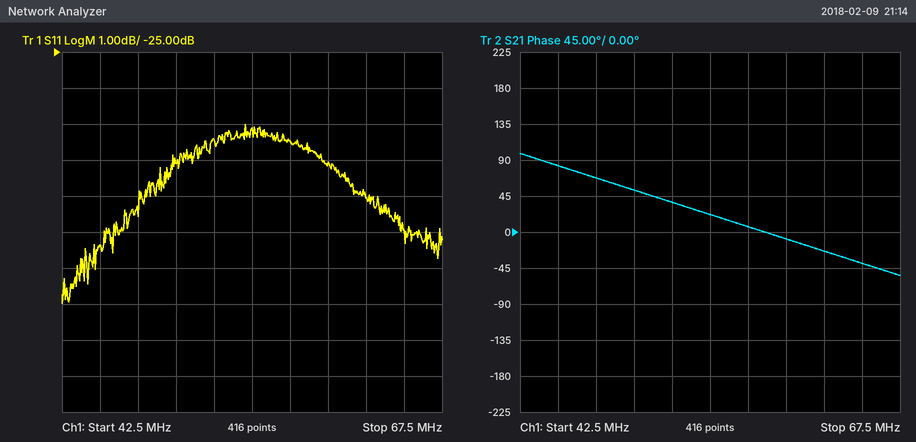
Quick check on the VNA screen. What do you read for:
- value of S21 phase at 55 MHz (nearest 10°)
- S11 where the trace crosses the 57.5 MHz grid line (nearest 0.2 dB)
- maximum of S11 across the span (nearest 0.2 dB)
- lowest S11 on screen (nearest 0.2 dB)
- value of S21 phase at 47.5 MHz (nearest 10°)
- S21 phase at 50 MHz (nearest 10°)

20°
-27.4 dB
-27.0 dB
-32.0 dB
70°
50°
